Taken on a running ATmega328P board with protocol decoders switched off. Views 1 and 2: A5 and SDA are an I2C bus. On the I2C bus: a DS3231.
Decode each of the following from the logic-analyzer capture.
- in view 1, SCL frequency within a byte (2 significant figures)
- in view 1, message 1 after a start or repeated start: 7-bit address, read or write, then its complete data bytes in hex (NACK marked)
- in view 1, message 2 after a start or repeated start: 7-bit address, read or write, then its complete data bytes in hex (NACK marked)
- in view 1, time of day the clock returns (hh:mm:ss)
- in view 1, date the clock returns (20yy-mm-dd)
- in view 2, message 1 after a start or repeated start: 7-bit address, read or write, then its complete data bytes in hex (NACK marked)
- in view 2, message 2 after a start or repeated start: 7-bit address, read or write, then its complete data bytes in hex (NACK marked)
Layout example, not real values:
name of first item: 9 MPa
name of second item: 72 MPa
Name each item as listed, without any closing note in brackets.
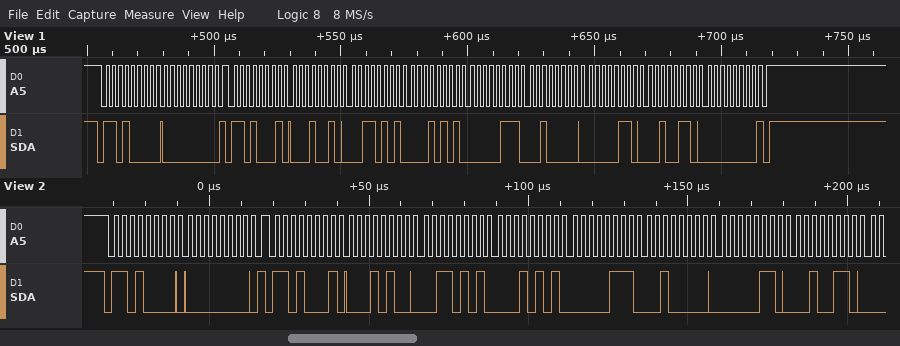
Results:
in view 1, SCL frequency within a byte: 400 kHz
in view 1, message 1 after a start or repeated start: 7-bit address, read or write, then its complete data bytes in hex: 0x68 write: 00
in view 1, message 2 after a start or repeated start: 7-bit address, read or write, then its complete data bytes in hex: 0x68 read: 12 35 15 07 20 06 26 00 NACK
in view 1, time of day the clock returns: 15:35:12
in view 1, date the clock returns: 2026-06-20
in view 2, message 1 after a start or repeated start: 7-bit address, read or write, then its complete data bytes in hex: 0x68 write: 00
in view 2, message 2 after a start or repeated start: 7-bit address, read or write, then its complete data bytes in hex: 0x68 read: 14 35 15 07 20 06 26
